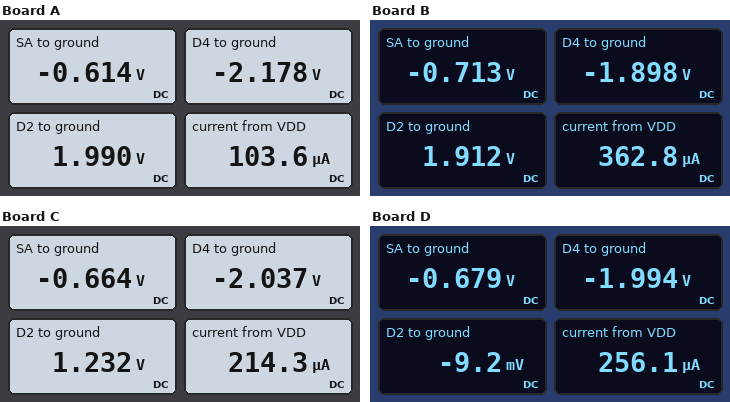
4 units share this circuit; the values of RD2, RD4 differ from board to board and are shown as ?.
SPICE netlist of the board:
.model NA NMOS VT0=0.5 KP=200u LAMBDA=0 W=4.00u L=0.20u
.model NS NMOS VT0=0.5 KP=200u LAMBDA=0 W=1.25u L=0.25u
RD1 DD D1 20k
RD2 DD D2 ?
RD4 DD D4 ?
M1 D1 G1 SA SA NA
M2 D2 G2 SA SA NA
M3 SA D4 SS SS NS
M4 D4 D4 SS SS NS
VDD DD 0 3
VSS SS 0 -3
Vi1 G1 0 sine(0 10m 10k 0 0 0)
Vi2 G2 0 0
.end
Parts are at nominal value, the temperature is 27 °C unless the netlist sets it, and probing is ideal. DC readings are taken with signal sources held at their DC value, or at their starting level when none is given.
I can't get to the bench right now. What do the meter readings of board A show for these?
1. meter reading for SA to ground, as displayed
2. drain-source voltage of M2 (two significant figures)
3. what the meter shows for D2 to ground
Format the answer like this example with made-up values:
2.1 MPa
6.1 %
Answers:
-0.614 V
2.6 V
1.990 V
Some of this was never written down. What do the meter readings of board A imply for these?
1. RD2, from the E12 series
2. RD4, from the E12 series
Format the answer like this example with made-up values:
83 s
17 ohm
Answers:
39 kΩ
100 kΩ
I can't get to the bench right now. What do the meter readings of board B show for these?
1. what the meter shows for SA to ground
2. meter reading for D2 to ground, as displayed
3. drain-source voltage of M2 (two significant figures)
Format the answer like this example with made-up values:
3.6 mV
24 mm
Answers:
-0.713 V
1.912 V
2.6 V
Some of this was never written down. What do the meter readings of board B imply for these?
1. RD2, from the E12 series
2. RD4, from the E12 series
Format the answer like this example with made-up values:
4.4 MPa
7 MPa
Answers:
12 kΩ
27 kΩ
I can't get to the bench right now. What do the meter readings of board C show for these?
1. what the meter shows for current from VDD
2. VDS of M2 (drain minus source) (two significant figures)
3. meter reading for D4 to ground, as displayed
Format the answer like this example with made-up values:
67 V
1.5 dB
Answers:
214.3 µA
1.9 V
-2.037 V
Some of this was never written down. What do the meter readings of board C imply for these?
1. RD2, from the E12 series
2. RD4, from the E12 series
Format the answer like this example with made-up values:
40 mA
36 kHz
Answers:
33 kΩ
47 kΩ
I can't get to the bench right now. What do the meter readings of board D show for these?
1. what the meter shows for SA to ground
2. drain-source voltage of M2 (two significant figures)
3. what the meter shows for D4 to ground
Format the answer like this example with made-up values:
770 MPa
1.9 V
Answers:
-0.679 V
670 mV
-1.994 V
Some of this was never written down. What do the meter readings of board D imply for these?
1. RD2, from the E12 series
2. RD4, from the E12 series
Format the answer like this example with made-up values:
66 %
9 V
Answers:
47 kΩ
39 kΩ
